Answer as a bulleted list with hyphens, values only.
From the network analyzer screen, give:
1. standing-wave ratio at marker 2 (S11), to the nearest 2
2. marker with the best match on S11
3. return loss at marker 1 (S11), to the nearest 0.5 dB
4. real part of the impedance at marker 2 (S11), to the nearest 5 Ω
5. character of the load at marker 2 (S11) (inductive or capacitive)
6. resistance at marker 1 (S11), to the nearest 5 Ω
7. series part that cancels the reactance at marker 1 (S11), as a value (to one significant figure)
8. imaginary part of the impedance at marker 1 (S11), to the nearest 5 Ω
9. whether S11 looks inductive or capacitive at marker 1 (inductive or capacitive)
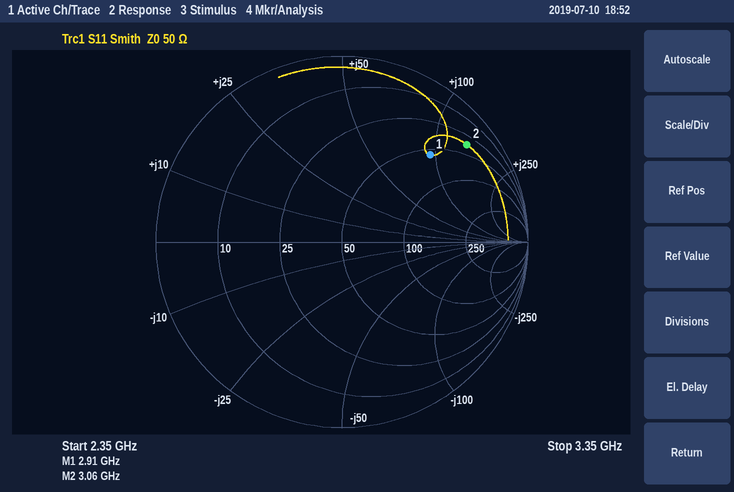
- 12
- marker 1
- 3.5 dB
- 35 Ω
- inductive
- 55 Ω
- 600 fF
- +95 Ω
- inductive
